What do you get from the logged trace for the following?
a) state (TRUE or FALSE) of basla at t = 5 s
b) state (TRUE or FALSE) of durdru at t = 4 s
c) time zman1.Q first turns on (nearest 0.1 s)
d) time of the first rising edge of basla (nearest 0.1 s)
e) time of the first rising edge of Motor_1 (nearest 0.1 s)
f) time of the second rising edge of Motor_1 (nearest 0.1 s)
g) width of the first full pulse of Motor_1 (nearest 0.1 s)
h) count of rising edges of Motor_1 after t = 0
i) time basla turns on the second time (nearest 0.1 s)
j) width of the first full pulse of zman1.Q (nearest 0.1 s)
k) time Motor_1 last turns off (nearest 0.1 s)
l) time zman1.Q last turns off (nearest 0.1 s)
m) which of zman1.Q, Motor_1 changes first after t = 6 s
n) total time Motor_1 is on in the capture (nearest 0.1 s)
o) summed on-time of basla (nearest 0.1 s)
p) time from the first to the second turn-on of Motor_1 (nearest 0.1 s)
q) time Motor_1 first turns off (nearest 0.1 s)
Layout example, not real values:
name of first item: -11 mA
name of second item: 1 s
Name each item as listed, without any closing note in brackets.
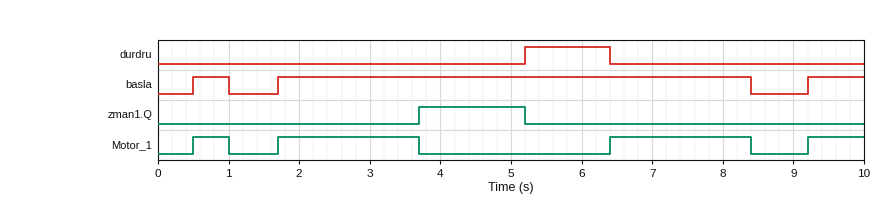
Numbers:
state (TRUE or FALSE) of basla at t = 5 s: TRUE
state (TRUE or FALSE) of durdru at t = 4 s: FALSE
time zman1.Q first turns on: 3.7 s
time of the first rising edge of basla: 0.5 s
time of the first rising edge of Motor_1: 0.5 s
time of the second rising edge of Motor_1: 1.7 s
width of the first full pulse of Motor_1: 0.5 s
count of rising edges of Motor_1 after t = 0: 4
time basla turns on the second time: 1.7 s
width of the first full pulse of zman1.Q: 1.5 s
time Motor_1 last turns off: 8.4 s
time zman1.Q last turns off: 5.2 s
which of zman1.Q, Motor_1 changes first after t = 6 s: Motor_1
total time Motor_1 is on in the capture: 5.3 s
summed on-time of basla: 8.0 s
time from the first to the second turn-on of Motor_1: 1.2 s
time Motor_1 first turns off: 1.0 s
